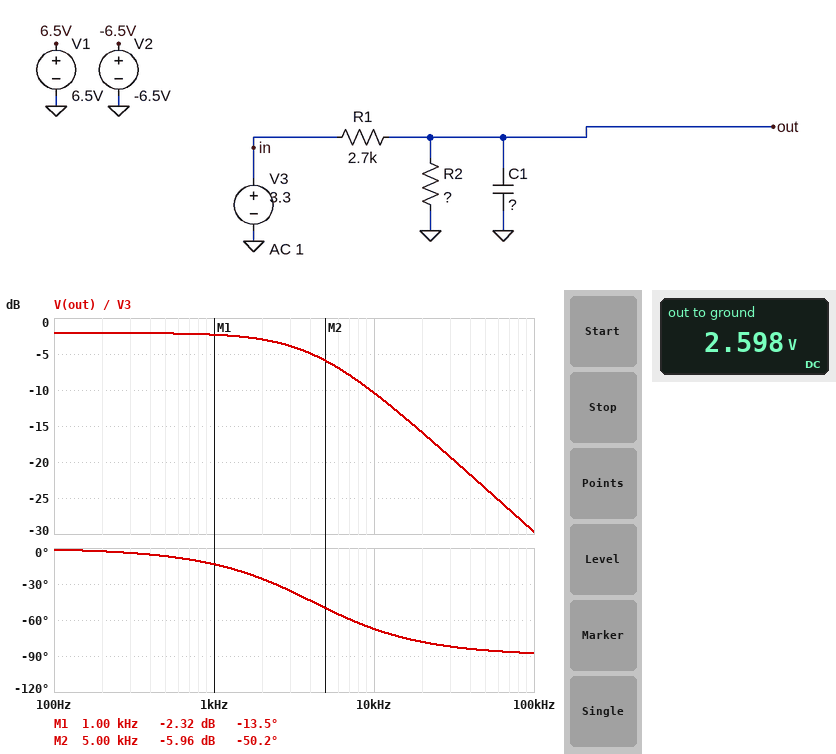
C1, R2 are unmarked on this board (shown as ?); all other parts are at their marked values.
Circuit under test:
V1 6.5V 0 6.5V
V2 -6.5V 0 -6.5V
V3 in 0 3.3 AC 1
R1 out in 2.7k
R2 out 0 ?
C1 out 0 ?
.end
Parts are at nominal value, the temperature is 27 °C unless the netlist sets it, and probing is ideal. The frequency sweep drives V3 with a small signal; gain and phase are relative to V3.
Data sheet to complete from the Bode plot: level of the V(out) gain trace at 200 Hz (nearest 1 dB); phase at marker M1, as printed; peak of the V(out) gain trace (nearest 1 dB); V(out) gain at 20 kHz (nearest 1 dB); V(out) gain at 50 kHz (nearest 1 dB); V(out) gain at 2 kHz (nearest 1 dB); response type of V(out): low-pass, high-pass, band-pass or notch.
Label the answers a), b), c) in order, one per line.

a) -2 dB
b) -13.5 deg
c) -2 dB
d) -16 dB
e) -24 dB
f) -3 dB
g) low-pass
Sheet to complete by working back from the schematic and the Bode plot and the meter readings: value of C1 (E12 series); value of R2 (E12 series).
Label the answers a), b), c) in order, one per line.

a) 18 nF
b) 10 kΩ
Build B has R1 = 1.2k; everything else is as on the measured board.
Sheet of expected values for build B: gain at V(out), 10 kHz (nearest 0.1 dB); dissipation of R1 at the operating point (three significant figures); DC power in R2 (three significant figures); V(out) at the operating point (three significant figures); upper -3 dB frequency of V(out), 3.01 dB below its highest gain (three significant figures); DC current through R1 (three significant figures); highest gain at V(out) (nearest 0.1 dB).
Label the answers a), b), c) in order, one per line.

a) -4.9 dB
b) 104 µW
c) 868 µW
d) 2.95 V
e) 8.25 kHz
f) 295 µA
g) -1.0 dB
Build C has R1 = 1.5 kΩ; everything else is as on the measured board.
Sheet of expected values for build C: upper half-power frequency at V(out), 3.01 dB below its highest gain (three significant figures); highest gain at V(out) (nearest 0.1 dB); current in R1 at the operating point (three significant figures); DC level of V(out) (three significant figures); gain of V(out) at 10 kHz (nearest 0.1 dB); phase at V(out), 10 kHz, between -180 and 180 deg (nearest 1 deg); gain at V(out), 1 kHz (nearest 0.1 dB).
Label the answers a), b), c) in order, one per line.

a) 6.78 kHz
b) -1.2 dB
c) 287 µA
d) 2.87 V
e) -6.2 dB
f) -56 deg
g) -1.3 dB
